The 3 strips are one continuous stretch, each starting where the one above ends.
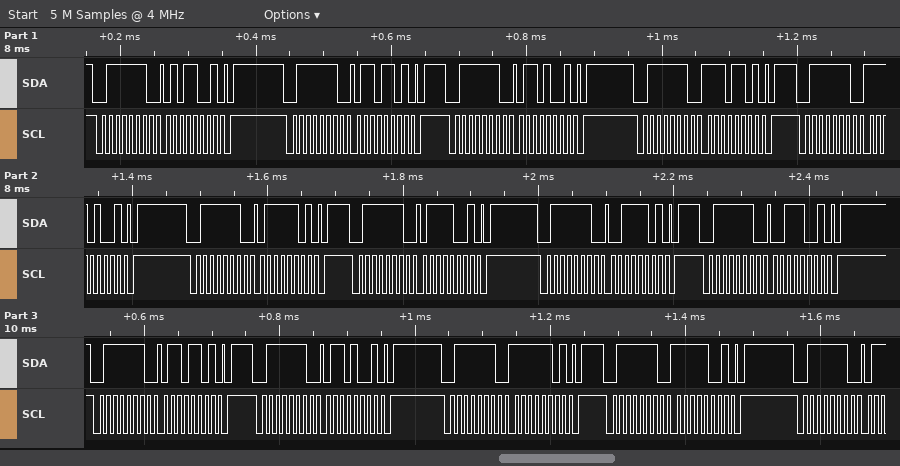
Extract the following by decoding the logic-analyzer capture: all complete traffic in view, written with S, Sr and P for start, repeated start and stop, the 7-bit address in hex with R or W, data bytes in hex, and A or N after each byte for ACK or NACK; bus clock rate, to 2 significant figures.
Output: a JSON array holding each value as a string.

["S 3FW A 59 A P S 3FW A 6D A P S 3FW A 69 A P S 3FW A ED A P S 3FW A E9 A P S 3FW A 7D A P S 3FW A 79 A P S 3FW A 3D A P S 3FW A 39 A P S 3FW A 6D A P S 3FW A 69 A P S 3FW A FD A P S 3FW A F9 A P S 3FW A", "100 kHz"]
